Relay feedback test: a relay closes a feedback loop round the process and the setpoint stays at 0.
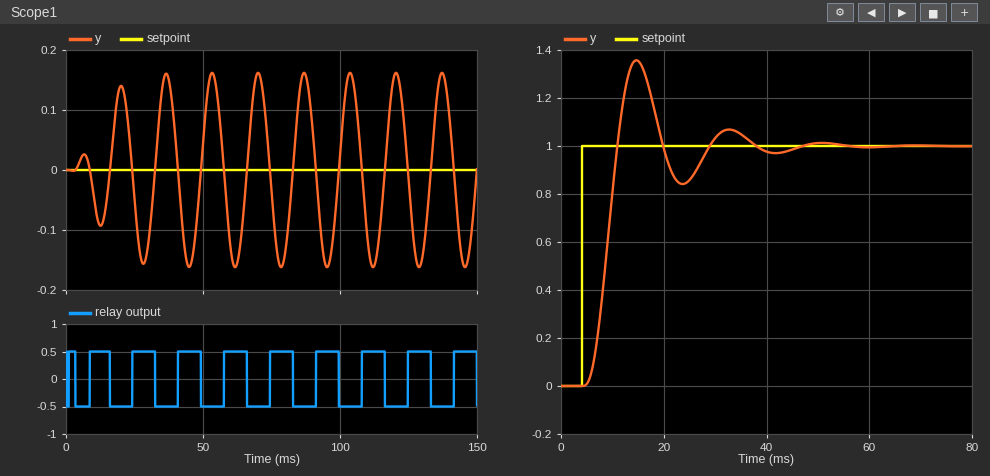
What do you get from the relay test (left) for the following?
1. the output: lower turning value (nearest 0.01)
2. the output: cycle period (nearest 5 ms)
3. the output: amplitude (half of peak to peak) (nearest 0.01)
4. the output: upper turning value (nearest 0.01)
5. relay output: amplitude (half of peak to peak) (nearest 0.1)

-0.16
15 ms
0.16
0.16
0.5
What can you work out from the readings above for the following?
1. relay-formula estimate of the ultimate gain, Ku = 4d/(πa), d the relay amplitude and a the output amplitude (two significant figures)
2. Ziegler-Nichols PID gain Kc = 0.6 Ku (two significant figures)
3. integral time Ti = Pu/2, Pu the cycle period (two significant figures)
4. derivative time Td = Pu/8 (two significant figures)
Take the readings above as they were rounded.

4.0
2.4
7.5 ms
1.9 ms
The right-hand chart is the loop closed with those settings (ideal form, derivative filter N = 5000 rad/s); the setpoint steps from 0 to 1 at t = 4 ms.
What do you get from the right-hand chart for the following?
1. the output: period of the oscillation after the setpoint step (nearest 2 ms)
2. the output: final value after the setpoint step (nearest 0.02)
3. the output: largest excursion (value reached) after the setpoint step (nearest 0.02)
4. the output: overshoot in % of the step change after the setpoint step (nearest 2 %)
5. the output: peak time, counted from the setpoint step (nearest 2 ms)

18 ms
1.00
1.36
36 %
10 ms
